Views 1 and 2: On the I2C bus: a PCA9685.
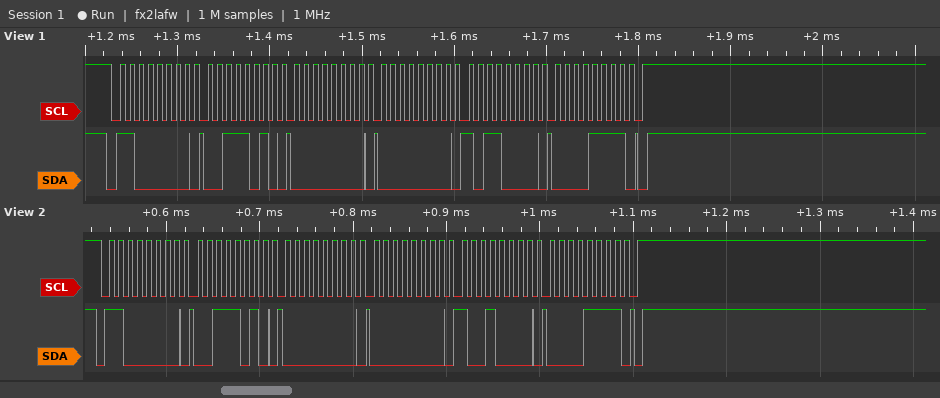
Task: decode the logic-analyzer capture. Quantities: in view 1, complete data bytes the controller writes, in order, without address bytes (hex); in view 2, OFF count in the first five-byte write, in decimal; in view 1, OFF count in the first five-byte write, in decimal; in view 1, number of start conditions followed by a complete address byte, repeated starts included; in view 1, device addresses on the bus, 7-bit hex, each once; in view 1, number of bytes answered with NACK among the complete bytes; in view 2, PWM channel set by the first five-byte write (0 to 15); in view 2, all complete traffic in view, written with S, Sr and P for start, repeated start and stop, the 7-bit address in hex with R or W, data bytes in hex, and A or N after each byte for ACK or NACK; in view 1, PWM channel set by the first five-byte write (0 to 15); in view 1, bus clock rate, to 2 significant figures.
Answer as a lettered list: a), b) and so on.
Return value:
a) 3A 00 00 B0 0F
b) 3984
c) 4016
d) 1
e) 0x60
f) 0
g) 13
h) S 60W A 3A A 00 A 00 A 90 A 0F A P
i) 13
j) 100 kHz
